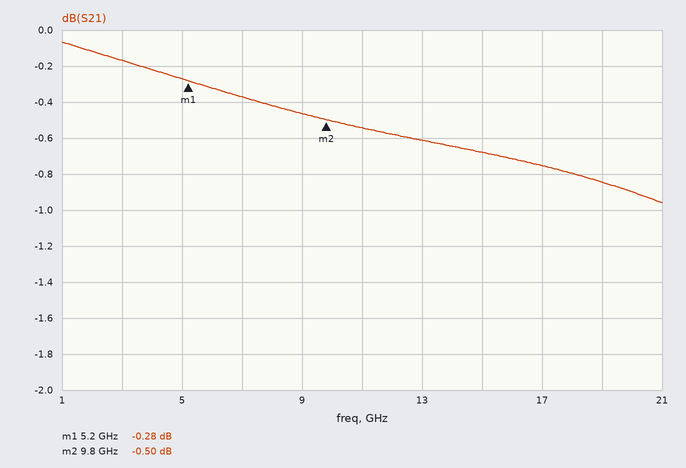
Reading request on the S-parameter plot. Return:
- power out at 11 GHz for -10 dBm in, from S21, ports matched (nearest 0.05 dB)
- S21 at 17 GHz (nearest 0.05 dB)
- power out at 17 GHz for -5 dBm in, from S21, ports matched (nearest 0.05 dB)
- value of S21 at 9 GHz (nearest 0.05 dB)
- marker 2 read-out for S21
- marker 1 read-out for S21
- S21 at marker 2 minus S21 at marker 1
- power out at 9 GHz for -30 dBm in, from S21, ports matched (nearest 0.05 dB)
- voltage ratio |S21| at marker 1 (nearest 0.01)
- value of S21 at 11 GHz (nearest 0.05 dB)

-10.55 dBm
-0.75 dB
-5.75 dBm
-0.45 dB
-0.50 dB
-0.28 dB
-0.22 dB
-30.45 dBm
0.97
-0.55 dB
